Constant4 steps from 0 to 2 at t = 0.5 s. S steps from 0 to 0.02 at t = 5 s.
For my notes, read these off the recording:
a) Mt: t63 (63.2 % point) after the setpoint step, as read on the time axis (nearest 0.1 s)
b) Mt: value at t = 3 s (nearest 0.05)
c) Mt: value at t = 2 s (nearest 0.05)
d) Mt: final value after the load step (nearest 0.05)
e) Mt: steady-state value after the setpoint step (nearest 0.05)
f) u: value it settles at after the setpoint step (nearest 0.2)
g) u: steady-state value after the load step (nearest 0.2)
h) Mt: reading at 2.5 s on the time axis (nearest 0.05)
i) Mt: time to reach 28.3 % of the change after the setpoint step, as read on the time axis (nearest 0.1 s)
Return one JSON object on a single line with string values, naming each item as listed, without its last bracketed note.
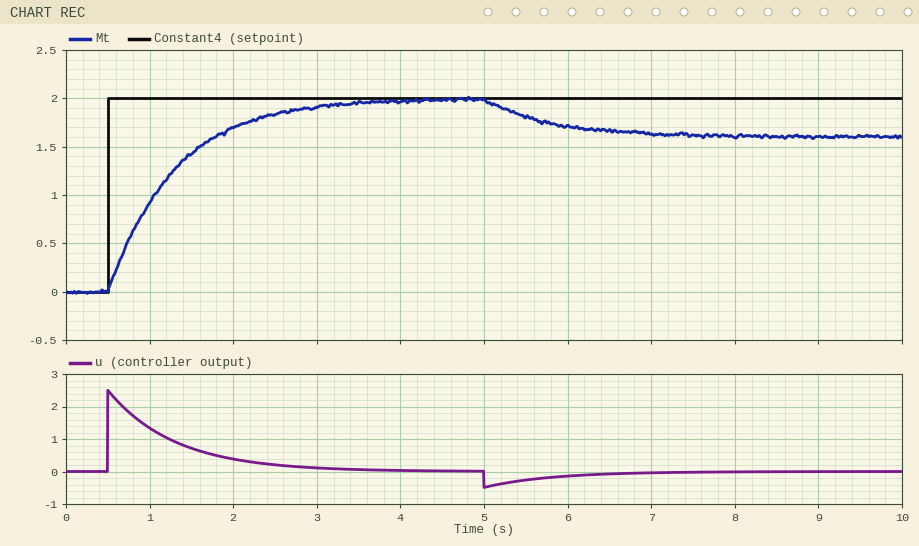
{"Mt: t63 (63.2 % point) after the setpoint step, as read on the time axis": "1.3 s", "Mt: value at t = 3 s": "1.90", "Mt: value at t = 2 s": "1.70", "Mt: final value after the load step": "1.60", "Mt: steady-state value after the setpoint step": "2.00", "u: value it settles at after the setpoint step": "0.0", "u: steady-state value after the load step": "0.0", "Mt: reading at 2.5 s on the time axis": "1.85", "Mt: time to reach 28.3 % of the change after the setpoint step, as read on the time axis": "0.8 s"}
